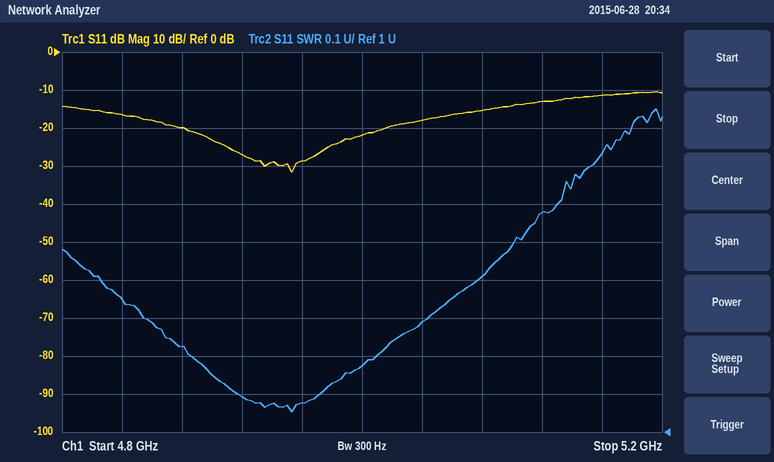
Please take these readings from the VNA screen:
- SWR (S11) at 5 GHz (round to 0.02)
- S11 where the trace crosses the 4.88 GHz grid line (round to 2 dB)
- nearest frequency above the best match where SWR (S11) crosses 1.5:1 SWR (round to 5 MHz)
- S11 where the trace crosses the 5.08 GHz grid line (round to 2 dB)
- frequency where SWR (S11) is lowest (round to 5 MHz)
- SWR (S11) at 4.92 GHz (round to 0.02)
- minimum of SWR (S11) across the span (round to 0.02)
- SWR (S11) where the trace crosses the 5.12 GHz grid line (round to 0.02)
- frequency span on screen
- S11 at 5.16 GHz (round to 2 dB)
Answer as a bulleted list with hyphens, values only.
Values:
- 1.18
- -20 dB
- 5.100 GHz
- -16 dB
- 4.955 GHz
- 1.10
- 1.06
- 1.58
- 400 MHz
- -12 dB
